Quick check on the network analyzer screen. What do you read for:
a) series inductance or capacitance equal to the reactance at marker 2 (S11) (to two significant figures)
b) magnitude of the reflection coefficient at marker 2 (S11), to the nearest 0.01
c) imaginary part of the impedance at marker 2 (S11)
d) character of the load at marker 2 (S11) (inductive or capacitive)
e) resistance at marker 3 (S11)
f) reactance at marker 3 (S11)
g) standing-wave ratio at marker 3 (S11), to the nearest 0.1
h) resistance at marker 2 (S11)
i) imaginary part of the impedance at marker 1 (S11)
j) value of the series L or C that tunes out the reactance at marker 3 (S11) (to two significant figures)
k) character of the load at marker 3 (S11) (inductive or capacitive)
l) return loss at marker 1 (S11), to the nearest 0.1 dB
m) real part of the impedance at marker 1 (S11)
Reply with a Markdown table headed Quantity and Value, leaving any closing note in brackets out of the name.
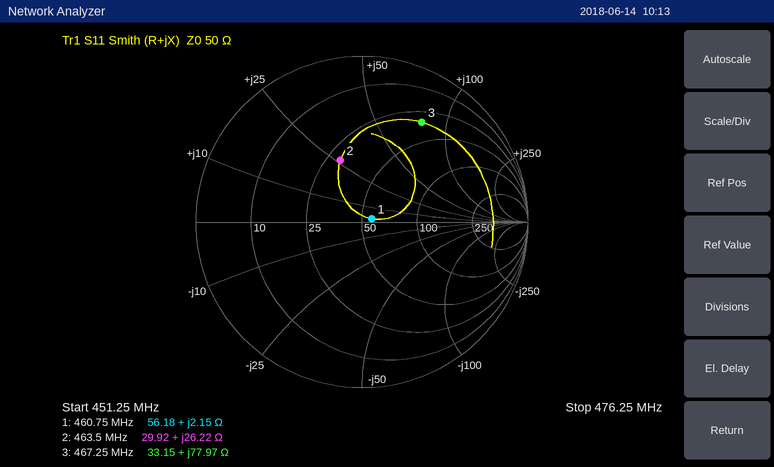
| Quantity | Value |
|---|---|
| series inductance or capacitance equal to the reactance at marker 2 (S11) | 9.0 nH |
| magnitude of the reflection coefficient at marker 2 (S11), to the nearest 0.01 | 0.39 |
| imaginary part of the impedance at marker 2 | +26.22 Ω |
| character of the load at marker 2 (S11) | inductive |
| resistance at marker 3 | 33.15 Ω |
| reactance at marker 3 | +77.97 Ω |
| standing-wave ratio at marker 3 (S11), to the nearest 0.1 | 5.7 |
| resistance at marker 2 | 29.92 Ω |
| imaginary part of the impedance at marker 1 | +2.15 Ω |
| value of the series L or C that tunes out the reactance at marker 3 (S11) | 4.4 pF |
| character of the load at marker 3 (S11) | inductive |
| return loss at marker 1 (S11), to the nearest 0.1 dB | 24.2 dB |
| real part of the impedance at marker 1 | 56.18 Ω |
